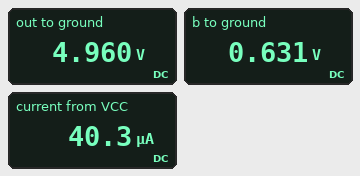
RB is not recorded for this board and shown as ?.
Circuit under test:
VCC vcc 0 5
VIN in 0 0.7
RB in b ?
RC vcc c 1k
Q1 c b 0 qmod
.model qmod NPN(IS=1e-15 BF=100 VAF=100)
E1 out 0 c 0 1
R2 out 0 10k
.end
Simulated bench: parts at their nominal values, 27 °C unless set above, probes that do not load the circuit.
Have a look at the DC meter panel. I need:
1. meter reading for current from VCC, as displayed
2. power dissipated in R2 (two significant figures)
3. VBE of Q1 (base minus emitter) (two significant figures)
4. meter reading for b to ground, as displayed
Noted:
40.3 µA
2.5 mW
630 mV
0.631 V
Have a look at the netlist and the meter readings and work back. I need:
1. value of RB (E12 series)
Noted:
180 kΩ
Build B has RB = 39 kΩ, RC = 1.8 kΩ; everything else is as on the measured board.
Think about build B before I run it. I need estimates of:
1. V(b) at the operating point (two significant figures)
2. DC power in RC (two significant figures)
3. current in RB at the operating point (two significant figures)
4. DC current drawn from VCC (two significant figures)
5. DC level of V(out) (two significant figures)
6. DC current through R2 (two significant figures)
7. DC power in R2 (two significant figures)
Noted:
660 mV
23 µW
1.1 µA
110 µA
4.8 V
480 µA
2.3 mW
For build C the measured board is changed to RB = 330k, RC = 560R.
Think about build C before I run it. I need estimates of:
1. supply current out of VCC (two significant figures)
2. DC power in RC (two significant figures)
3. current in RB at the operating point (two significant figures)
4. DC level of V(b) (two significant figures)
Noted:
26 µA
370 nW
250 nA
620 mV
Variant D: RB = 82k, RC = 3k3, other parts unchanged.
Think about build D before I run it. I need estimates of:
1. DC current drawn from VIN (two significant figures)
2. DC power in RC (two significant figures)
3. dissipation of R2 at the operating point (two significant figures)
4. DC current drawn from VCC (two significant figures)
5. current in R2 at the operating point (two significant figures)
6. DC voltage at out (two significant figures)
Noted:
670 nA
16 µW
2.3 mW
70 µA
480 µA
4.8 V
